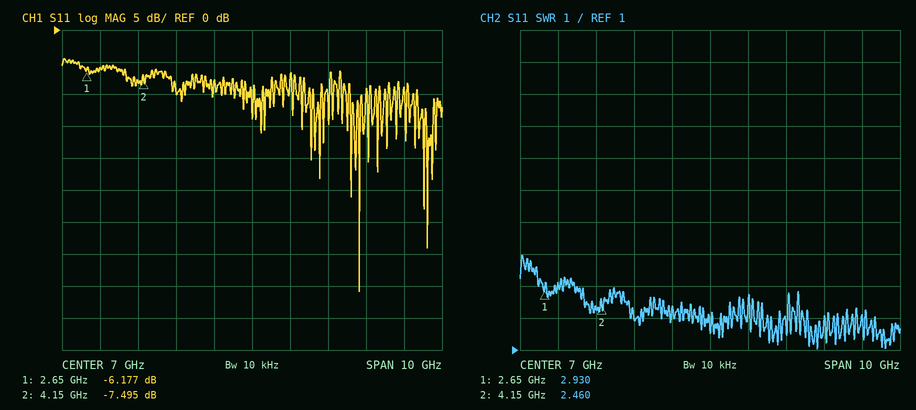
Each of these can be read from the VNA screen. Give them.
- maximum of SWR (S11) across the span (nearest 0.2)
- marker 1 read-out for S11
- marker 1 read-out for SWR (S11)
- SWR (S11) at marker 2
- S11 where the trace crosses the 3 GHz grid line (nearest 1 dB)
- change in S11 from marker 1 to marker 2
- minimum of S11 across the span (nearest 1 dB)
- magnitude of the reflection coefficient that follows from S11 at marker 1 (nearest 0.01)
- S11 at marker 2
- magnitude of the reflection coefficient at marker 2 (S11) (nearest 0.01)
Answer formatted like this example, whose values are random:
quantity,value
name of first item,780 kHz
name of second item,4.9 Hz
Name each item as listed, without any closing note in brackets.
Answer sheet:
quantity,value
maximum of SWR (S11) across the span,4.0
marker 1 read-out for S11,-6.177 dB
marker 1 read-out for SWR,2.930
SWR (S11) at marker 2,2.460
S11 where the trace crosses the 3 GHz grid line,-6 dB
change in S11 from marker 1 to marker 2,-1.318 dB
minimum of S11 across the span,-41 dB
magnitude of the reflection coefficient that follows from S11 at marker 1,0.49
S11 at marker 2,-7.495 dB
magnitude of the reflection coefficient at marker 2 (S11),0.42
